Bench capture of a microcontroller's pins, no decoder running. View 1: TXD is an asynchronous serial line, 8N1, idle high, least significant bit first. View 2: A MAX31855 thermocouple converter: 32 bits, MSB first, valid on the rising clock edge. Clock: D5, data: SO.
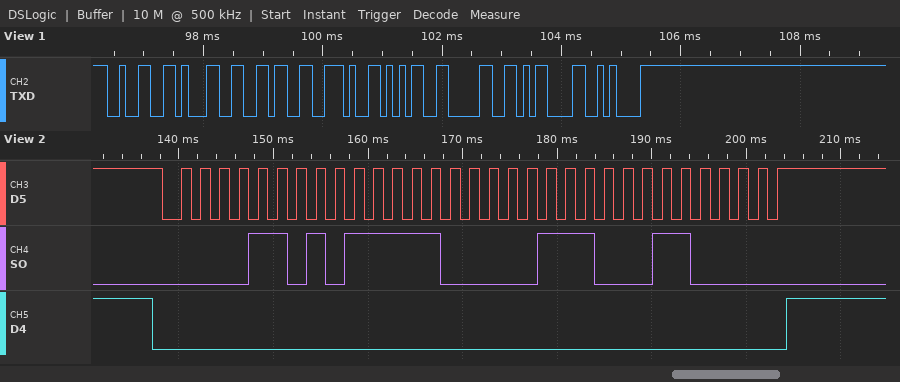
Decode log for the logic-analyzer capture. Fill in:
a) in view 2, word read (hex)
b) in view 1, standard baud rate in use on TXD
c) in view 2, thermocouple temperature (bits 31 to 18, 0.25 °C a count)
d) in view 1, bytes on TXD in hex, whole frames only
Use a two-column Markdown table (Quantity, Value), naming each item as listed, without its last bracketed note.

| Quantity | Value |
|---|---|
| in view 2, word read | 0x0D7C1C60 |
| in view 1, standard baud rate in use on TXD | 9600 baud |
| in view 2, thermocouple temperature | 215.75 °C |
| in view 1, bytes on TXD in hex, whole frames only | 32 31 36 2E 35 30 0D 0A |
